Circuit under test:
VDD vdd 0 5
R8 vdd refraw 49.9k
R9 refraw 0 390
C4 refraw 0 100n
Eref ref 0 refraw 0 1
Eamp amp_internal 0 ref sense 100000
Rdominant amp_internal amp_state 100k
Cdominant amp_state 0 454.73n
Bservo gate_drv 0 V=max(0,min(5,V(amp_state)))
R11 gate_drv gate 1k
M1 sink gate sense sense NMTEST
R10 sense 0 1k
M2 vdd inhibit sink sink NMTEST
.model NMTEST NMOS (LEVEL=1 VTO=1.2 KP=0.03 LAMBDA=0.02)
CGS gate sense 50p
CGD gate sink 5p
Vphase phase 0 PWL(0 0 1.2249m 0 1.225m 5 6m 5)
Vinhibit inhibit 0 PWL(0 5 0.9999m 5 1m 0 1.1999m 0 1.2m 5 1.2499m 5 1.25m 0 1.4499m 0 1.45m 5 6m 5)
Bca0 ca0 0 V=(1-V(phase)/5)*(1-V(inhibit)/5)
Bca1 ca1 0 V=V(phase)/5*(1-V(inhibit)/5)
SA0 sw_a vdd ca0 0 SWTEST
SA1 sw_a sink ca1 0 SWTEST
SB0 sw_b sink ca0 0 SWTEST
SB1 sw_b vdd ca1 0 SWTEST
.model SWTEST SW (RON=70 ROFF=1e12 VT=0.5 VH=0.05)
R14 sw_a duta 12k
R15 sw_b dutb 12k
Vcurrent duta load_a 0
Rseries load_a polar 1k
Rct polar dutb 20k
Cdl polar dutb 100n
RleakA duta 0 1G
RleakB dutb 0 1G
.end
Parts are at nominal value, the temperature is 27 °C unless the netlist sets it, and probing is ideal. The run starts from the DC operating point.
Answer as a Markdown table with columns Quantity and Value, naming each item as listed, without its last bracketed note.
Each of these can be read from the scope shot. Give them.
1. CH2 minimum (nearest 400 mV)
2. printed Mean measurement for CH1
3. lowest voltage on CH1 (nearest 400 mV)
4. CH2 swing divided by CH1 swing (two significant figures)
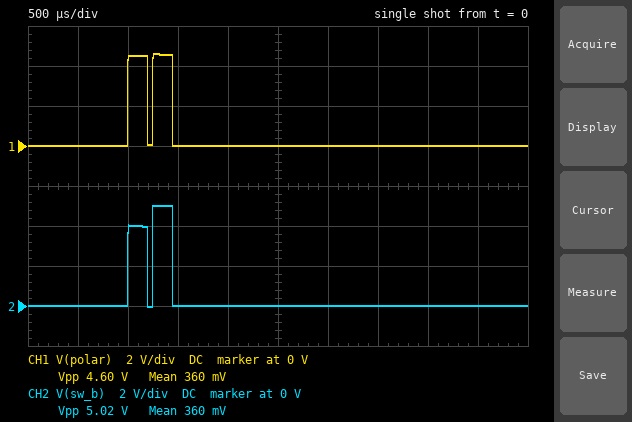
| Quantity | Value |
|---|---|
| CH2 minimum | 0 V |
| printed Mean measurement for CH1 | 360 mV |
| lowest voltage on CH1 | 0 V |
| CH2 swing divided by CH1 swing | 1.1 |
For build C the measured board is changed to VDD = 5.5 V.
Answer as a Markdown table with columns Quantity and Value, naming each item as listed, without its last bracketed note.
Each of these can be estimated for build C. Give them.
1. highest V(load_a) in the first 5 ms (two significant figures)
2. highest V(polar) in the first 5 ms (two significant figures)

| Quantity | Value |
|---|---|
| highest V(load_a) in the first 5 ms | 5.0 V |
| highest V(polar) in the first 5 ms | 5.1 V |
